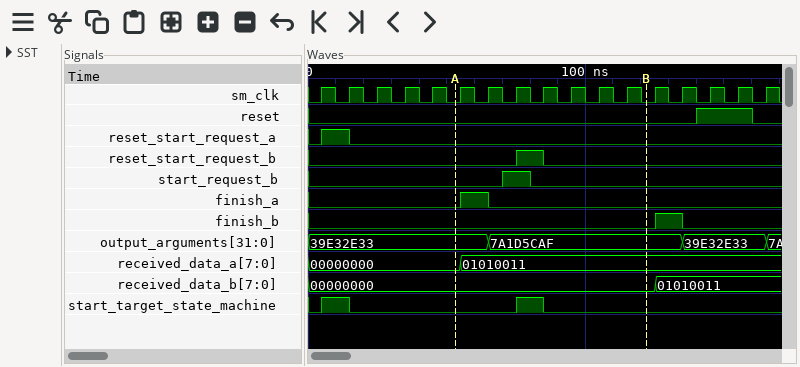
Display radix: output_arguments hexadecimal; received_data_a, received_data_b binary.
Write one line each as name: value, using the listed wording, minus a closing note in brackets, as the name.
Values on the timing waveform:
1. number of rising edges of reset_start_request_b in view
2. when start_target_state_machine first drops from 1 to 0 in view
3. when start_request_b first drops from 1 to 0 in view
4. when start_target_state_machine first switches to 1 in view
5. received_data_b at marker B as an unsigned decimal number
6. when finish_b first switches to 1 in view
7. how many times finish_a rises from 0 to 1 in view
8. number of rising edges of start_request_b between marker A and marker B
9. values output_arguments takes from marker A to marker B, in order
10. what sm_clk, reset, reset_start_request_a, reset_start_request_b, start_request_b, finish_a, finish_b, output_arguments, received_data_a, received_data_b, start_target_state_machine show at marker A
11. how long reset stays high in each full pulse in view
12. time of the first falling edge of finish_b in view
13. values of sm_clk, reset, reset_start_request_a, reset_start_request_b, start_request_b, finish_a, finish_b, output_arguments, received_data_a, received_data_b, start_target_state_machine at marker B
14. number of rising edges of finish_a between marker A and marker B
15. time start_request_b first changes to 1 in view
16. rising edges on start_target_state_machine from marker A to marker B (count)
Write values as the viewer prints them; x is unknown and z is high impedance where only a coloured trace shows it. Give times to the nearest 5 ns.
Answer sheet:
number of rising edges of reset_start_request_b in view: 1
when start_target_state_machine first drops from 1 to 0 in view: 15 ns
when start_request_b first drops from 1 to 0 in view: 80 ns
when start_target_state_machine first switches to 1 in view: 5 ns
received_data_b at marker B as an unsigned decimal number: 0
when finish_b first switches to 1 in view: 125 ns
how many times finish_a rises from 0 to 1 in view: 1
number of rising edges of start_request_b between marker A and marker B: 1
values output_arguments takes from marker A to marker B, in order: 39E32E33, 7A1D5CAF
what sm_clk, reset, reset_start_request_a, reset_start_request_b, start_request_b, finish_a, finish_b, output_arguments, received_data_a, received_data_b, start_target_state_machine show at marker A: sm_clk=0, reset=0, reset_start_request_a=0, reset_start_request_b=0, start_request_b=0, finish_a=0, finish_b=0, output_arguments=39E32E33, received_data_a=00000000, received_data_b=00000000, start_target_state_machine=0
how long reset stays high in each full pulse in view: 20 ns
time of the first falling edge of finish_b in view: 135 ns
values of sm_clk, reset, reset_start_request_a, reset_start_request_b, start_request_b, finish_a, finish_b, output_arguments, received_data_a, received_data_b, start_target_state_machine at marker B: sm_clk=0, reset=0, reset_start_request_a=0, reset_start_request_b=0, start_request_b=0, finish_a=0, finish_b=0, output_arguments=7A1D5CAF, received_data_a=01010011, received_data_b=00000000, start_target_state_machine=0
number of rising edges of finish_a between marker A and marker B: 1
time start_request_b first changes to 1 in view: 70 ns
rising edges on start_target_state_machine from marker A to marker B: 1
